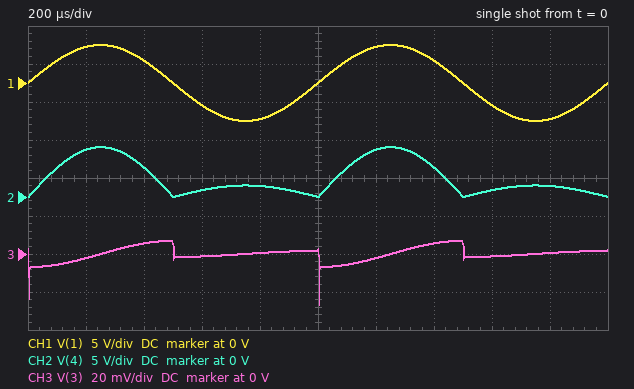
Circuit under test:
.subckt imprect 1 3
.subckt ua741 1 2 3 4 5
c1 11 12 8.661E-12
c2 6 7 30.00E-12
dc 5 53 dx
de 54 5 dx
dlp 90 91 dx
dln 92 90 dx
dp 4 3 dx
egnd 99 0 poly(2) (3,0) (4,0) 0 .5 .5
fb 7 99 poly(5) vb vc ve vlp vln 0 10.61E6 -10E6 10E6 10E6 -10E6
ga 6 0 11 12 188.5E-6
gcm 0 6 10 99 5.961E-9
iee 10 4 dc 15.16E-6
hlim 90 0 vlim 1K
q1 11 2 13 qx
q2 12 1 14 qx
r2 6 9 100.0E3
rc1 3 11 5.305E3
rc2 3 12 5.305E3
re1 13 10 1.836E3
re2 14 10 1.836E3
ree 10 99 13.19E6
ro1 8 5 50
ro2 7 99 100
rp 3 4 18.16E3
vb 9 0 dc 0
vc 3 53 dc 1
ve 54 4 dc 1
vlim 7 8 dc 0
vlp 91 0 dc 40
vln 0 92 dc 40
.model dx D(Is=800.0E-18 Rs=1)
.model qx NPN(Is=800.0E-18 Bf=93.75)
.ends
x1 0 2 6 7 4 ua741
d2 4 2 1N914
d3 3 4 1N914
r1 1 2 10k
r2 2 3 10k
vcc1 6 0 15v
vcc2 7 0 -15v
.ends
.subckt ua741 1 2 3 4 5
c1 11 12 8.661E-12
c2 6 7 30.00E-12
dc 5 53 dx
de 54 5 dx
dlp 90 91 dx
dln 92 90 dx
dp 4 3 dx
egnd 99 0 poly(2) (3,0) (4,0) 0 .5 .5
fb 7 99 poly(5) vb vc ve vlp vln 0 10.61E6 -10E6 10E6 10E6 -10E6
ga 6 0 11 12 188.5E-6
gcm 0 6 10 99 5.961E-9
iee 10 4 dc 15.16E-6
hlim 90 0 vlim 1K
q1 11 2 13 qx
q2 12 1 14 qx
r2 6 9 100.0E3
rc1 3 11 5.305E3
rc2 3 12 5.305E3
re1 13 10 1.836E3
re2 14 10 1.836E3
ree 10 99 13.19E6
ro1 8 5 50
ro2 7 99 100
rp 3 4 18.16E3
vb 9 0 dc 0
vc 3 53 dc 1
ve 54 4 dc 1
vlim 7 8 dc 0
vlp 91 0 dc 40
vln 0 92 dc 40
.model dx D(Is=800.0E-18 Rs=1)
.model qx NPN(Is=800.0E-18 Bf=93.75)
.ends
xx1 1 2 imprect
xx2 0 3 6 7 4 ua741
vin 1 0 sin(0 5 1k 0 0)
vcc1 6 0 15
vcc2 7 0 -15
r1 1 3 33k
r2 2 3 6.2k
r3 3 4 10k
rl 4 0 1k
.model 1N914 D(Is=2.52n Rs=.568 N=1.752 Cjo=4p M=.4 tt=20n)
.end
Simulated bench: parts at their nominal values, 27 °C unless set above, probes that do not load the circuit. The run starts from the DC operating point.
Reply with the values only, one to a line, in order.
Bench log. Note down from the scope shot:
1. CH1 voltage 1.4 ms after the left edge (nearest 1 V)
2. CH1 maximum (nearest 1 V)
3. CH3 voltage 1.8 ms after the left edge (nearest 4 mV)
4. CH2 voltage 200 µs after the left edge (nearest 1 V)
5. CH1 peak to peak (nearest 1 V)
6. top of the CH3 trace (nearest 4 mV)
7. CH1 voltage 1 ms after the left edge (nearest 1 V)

3 V
5 V
0 V
6 V
10 V
8 mV
0 V
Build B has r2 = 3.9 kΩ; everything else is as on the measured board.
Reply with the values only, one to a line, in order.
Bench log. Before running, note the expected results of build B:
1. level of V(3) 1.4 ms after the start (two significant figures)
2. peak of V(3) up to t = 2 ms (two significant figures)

9.6 mV
12 mV
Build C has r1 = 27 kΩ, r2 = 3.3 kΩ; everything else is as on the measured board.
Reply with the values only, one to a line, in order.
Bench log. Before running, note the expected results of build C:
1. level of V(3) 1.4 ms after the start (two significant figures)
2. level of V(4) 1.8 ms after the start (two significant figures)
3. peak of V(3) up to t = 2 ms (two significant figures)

11 mV
1.8 V
14 mV
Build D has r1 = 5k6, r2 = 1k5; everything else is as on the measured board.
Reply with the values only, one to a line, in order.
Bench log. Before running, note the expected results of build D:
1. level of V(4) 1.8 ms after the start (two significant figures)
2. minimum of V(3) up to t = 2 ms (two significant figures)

8.5 V
-1.0 V
